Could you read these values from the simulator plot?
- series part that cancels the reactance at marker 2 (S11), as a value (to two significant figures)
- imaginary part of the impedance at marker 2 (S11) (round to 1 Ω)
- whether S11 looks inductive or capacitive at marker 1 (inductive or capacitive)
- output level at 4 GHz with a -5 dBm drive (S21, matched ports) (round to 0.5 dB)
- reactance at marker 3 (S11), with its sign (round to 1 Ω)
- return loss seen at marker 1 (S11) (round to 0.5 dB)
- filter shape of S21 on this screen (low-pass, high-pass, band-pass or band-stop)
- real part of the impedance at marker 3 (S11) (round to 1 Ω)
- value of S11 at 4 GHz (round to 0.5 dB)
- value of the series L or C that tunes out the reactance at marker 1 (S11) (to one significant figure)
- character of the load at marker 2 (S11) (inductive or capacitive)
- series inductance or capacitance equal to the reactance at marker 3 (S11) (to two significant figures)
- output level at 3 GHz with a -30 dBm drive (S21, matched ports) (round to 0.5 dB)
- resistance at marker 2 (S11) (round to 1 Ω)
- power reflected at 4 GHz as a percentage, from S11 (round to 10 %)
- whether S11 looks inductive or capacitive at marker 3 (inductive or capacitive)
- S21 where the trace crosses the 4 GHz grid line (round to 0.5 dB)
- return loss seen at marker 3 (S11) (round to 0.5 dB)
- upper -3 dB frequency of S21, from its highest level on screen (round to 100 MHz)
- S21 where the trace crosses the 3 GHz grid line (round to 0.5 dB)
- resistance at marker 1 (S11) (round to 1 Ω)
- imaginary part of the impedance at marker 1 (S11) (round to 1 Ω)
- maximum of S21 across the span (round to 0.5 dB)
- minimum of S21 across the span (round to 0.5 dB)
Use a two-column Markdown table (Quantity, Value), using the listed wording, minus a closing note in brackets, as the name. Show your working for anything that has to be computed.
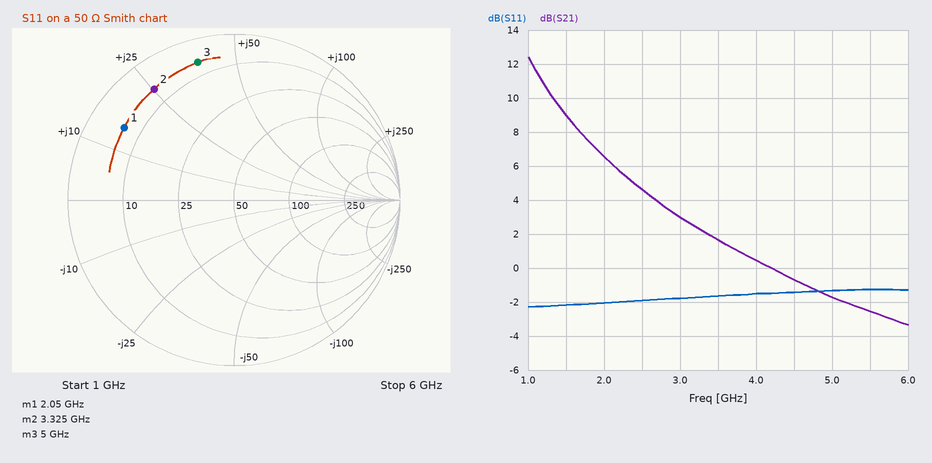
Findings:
| Quantity | Value |
|---|---|
| series part that cancels the reactance at marker 2 (S11), as a value | C = 1/(2π × 3.325 GHz × 25 Ω) ≈ 1.9 pF |
| imaginary part of the impedance at marker 2 (S11) | +25 Ω |
| whether S11 looks inductive or capacitive at marker 1 | inductive |
| output level at 4 GHz with a -5 dBm drive (S21, matched ports) | -5 dBm + (0.5 dB) = -4.5 dBm |
| reactance at marker 3 (S11), with its sign | +38 Ω |
| return loss seen at marker 1 (S11) | 2.0 dB |
| filter shape of S21 on this screen | low-pass |
| real part of the impedance at marker 3 (S11) | 6 Ω |
| value of S11 at 4 GHz | -1.5 dB |
| value of the series L or C that tunes out the reactance at marker 1 (S11) | C = 1/(2π × 2.05 GHz × 15 Ω) ≈ 5 pF |
| character of the load at marker 2 (S11) | inductive |
| series inductance or capacitance equal to the reactance at marker 3 (S11) | L = 38 Ω/(2π × 5 GHz) ≈ 1.2 nH |
| output level at 3 GHz with a -30 dBm drive (S21, matched ports) | -30 dBm + (3.0 dB) = -27.0 dBm |
| resistance at marker 2 (S11) | 6 Ω |
| power reflected at 4 GHz as a percentage, from S11 | 10^(-1.5/10) ≈ 70.8 %, so 70 % to the nearest 10 % |
| whether S11 looks inductive or capacitive at marker 3 | inductive |
| S21 where the trace crosses the 4 GHz grid line | 0.5 dB |
| return loss seen at marker 3 (S11) | 1.5 dB |
| upper -3 dB frequency of S21, from its highest level on screen | 1.4 GHz |
| S21 where the trace crosses the 3 GHz grid line | 3.0 dB |
| resistance at marker 1 (S11) | 6 Ω |
| imaginary part of the impedance at marker 1 (S11) | +15 Ω |
| maximum of S21 across the span | 12.5 dB |
| minimum of S21 across the span | -3.5 dB |
